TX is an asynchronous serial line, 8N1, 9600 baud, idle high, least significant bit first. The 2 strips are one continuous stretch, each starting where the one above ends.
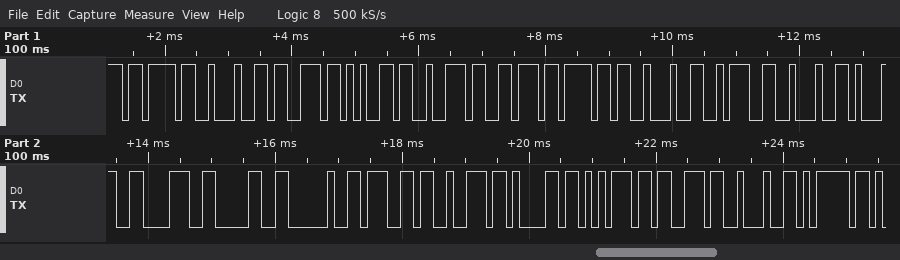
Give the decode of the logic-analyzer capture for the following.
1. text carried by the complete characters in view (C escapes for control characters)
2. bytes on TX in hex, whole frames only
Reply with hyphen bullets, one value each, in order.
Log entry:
- "{\"servo\":\"180 graus\"}"
- 7B 22 73 65 72 76 6F 22 3A 22 31 38 30 20 67 72 61 75 73 22 7D
